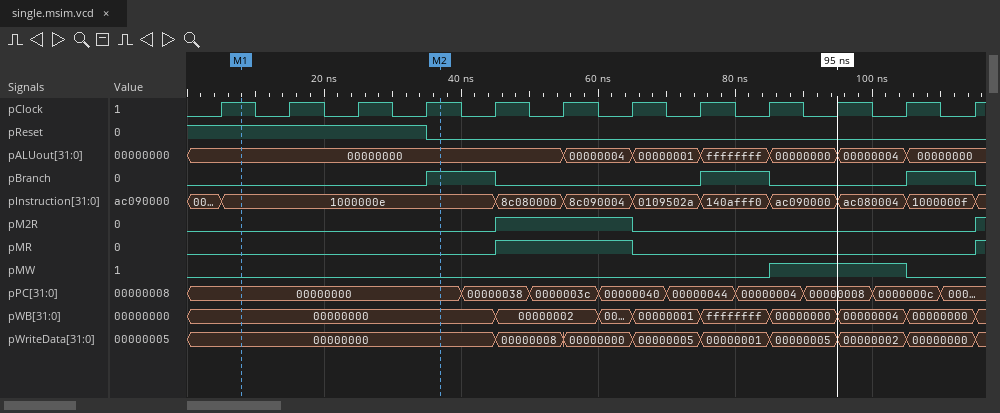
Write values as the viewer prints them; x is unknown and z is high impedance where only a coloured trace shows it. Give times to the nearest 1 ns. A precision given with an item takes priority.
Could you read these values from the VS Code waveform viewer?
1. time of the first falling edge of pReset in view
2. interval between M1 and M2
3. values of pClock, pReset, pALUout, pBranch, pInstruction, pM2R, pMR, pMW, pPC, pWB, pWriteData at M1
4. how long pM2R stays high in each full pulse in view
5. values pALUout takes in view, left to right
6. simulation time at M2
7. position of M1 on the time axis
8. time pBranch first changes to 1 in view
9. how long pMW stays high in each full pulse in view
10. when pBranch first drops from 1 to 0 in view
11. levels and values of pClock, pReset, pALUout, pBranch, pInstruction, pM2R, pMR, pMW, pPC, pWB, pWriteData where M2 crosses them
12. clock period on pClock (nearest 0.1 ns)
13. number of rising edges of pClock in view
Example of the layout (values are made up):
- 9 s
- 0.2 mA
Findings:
- 35 ns
- 29 ns
- pClock=1, pReset=1, pALUout=00000000, pBranch=0, pInstruction=1000000e, pM2R=0, pMR=0, pMW=0, pPC=00000000, pWB=00000000, pWriteData=00000000
- 20 ns
- 00000000, 00000004, 00000001, ffffffff, 00000000, 00000004, 00000000
- 37 ns
- 8 ns
- 35 ns
- 20 ns
- 45 ns
- pClock=1, pReset=0, pALUout=00000000, pBranch=1, pInstruction=1000000e, pM2R=0, pMR=0, pMW=0, pPC=00000000, pWB=00000000, pWriteData=00000000
- 10 ns
- 12
